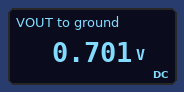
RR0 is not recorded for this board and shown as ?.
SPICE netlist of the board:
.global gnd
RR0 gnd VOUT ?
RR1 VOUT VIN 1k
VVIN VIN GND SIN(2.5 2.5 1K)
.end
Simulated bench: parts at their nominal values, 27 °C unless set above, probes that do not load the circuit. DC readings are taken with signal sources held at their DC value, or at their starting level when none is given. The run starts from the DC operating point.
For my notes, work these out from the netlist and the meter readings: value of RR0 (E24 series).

390 Ω
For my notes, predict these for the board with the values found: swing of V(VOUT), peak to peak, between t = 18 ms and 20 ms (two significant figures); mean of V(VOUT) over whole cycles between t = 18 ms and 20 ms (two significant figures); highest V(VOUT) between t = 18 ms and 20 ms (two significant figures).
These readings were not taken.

1.4 V
700 mV
1.4 V
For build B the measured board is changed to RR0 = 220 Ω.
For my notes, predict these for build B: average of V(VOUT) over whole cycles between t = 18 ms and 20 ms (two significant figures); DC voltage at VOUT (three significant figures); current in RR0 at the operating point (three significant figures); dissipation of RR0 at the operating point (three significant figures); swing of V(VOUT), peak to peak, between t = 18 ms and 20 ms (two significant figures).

450 mV
451 mV
2.05 mA
924 µW
900 mV
